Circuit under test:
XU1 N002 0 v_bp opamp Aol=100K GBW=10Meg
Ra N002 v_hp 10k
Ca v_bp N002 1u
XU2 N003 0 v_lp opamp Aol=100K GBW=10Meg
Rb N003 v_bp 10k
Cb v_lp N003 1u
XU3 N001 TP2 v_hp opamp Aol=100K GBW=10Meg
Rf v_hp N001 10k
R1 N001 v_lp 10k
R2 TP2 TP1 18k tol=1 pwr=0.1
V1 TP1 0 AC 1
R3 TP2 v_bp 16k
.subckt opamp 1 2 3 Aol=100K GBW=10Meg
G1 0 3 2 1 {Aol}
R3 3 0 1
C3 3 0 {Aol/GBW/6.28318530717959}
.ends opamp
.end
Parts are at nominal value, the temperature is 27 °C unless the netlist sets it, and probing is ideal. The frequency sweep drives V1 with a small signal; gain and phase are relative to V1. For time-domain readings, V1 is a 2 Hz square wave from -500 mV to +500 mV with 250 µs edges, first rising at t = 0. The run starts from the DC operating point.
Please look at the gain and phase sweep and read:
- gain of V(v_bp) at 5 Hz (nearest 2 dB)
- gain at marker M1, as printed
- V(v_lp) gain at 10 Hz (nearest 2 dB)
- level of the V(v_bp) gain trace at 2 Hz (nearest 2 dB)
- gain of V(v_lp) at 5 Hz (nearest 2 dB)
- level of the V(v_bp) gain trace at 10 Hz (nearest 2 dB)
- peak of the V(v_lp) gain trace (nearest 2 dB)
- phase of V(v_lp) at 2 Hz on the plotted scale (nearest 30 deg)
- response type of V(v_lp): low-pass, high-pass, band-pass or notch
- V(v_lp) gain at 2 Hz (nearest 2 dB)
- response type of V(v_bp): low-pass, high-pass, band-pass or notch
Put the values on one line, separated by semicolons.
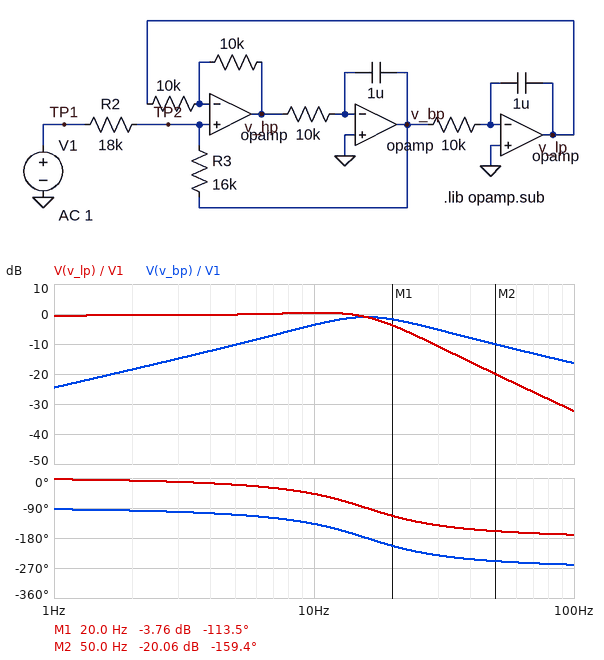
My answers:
-10 dB; -3.76 dB; 0 dB; -18 dB; 0 dB; -4 dB; 0 dB; 0 deg; low-pass; 0 dB; band-pass
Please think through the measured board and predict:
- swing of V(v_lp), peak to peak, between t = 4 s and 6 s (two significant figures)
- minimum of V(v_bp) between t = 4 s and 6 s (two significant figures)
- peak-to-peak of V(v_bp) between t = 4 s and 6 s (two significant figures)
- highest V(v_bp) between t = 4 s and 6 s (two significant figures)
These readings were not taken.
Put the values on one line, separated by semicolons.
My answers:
1.2 V; -500 mV; 1.0 V; 500 mV
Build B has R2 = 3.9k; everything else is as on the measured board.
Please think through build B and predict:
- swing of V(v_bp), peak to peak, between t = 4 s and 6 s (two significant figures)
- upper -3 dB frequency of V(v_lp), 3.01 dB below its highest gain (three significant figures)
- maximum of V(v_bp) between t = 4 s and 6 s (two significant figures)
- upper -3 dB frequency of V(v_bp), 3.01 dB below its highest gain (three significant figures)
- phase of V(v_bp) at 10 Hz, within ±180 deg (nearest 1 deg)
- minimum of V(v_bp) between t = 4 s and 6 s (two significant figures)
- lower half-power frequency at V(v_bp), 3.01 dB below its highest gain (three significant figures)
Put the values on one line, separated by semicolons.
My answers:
2.4 V; 18.2 Hz; 1.2 V; 19.3 Hz; -112 deg; -1.2 V; 13.1 Hz
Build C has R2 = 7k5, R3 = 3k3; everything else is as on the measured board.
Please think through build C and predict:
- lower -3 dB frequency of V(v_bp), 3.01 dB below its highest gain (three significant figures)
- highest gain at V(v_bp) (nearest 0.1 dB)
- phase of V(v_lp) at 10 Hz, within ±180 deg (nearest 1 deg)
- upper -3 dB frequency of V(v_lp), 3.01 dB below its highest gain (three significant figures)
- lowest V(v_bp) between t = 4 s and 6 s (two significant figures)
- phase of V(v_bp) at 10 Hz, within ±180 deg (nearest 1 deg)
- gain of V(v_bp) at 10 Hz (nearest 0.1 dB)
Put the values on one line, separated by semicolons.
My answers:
8.32 Hz; -7.1 dB; -55 deg; 16.2 Hz; -280 mV; -145 deg; -8.8 dB
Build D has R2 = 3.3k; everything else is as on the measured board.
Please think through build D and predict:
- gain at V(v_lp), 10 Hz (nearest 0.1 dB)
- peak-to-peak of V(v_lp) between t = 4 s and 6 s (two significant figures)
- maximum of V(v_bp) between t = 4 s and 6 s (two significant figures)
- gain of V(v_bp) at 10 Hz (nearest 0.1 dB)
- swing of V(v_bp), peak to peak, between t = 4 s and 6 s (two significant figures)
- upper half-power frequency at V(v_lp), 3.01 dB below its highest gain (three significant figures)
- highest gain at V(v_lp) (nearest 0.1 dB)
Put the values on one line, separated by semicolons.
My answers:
8.2 dB; 3.6 V; 1.3 V; 4.2 dB; 2.6 V; 18.0 Hz; 13.8 dB
